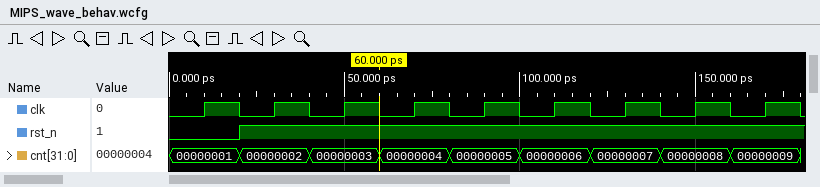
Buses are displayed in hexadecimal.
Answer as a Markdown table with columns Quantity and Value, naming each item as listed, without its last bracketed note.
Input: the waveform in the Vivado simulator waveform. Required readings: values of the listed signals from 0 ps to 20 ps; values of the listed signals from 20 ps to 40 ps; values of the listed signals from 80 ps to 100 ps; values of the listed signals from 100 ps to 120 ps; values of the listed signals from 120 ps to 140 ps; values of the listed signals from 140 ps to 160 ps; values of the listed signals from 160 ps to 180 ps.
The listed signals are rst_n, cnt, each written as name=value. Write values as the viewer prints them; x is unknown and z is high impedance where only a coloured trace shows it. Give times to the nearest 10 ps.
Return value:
| Quantity | Value |
|---|---|
| values of the listed signals from 0 ps to 20 ps | rst_n=0, cnt=00000001 |
| values of the listed signals from 20 ps to 40 ps | rst_n=1, cnt=00000002 |
| values of the listed signals from 80 ps to 100 ps | rst_n=1, cnt=00000005 |
| values of the listed signals from 100 ps to 120 ps | rst_n=1, cnt=00000006 |
| values of the listed signals from 120 ps to 140 ps | rst_n=1, cnt=00000007 |
| values of the listed signals from 140 ps to 160 ps | rst_n=1, cnt=00000008 |
| values of the listed signals from 160 ps to 180 ps | rst_n=1, cnt=00000009 |
